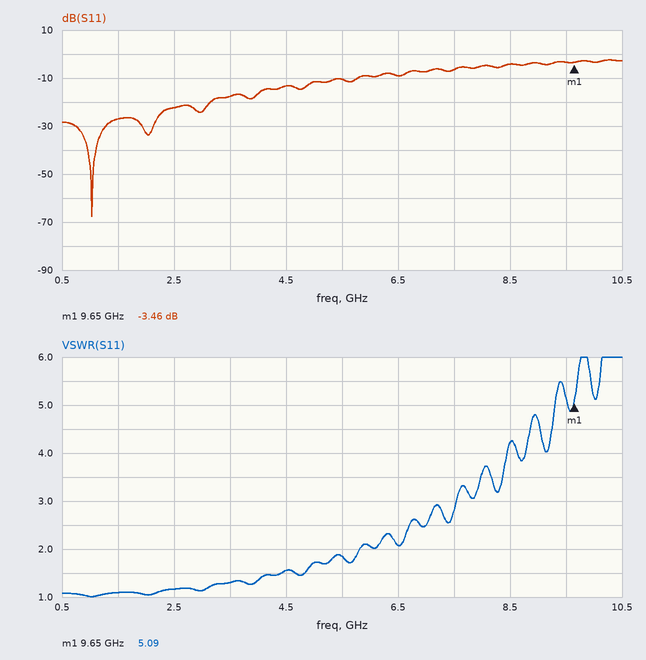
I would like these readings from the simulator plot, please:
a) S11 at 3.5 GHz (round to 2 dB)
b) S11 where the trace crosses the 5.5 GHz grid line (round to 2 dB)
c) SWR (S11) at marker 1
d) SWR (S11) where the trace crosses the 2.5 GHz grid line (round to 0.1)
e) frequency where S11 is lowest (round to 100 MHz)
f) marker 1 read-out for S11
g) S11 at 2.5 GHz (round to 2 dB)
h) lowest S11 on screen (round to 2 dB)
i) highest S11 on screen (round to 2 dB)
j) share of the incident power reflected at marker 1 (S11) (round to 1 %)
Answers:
-18 dB
-10 dB
5.09
1.2
1.0 GHz
-3.46 dB
-22 dB
-68 dB
-2 dB
45 %
